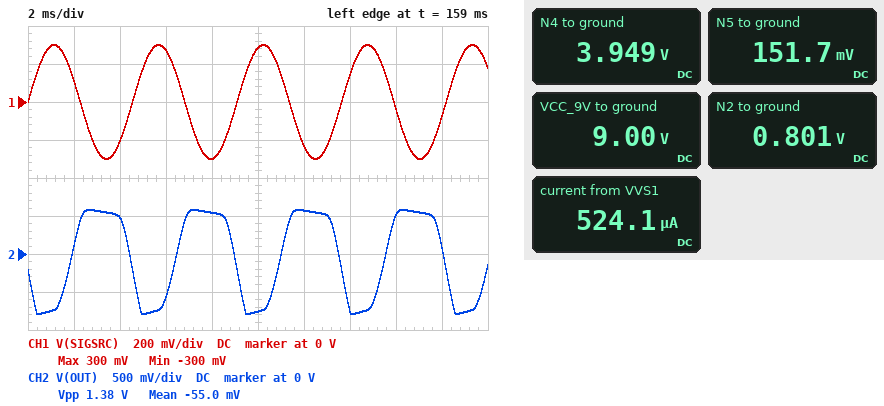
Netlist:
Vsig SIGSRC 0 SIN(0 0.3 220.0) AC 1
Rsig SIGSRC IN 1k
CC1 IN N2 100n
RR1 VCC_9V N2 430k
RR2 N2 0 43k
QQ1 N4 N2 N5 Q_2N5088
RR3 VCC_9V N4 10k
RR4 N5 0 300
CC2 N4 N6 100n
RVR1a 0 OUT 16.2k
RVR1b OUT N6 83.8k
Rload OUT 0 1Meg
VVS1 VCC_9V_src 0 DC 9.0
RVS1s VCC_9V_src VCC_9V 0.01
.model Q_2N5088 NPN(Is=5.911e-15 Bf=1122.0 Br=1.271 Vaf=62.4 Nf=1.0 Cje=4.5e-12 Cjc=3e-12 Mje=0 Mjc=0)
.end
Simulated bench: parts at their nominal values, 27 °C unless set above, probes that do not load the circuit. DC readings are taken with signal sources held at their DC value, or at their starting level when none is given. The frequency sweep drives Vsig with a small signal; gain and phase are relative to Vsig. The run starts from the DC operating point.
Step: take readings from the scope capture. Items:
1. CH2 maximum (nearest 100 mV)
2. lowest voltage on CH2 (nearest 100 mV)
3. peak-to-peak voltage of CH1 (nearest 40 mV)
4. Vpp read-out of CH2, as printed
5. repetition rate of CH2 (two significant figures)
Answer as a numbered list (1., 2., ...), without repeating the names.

1. 600 mV
2. -800 mV
3. 600 mV
4. 1.38 V
5. 220 Hz
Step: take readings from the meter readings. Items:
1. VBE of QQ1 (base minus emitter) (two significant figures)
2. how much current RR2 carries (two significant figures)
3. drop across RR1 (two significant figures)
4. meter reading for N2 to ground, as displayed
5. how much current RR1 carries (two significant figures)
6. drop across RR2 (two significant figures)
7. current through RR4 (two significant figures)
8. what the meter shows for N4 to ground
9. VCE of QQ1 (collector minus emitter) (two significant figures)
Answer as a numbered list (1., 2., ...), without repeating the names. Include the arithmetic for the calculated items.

1. 801 mV - 151.7 mV = 650 mV
2. (801 mV) / 43 kΩ = 19 µA
3. 9 V - 801 mV = 8.2 V
4. 0.801 V
5. (9 V - 801 mV) / 430 kΩ = 19 µA
6. 801 mV = 800 mV
7. (151.7 mV) / 300 Ω = 510 µA
8. 3.949 V
9. 3.949 V - 151.7 mV = 3.8 V
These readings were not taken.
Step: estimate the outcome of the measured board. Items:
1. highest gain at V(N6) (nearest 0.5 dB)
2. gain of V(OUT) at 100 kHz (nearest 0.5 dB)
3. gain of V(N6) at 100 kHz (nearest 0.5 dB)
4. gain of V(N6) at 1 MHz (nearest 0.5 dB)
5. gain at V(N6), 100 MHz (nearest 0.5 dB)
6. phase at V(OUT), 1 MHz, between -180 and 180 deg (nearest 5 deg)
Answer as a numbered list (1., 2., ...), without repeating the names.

1. 28.0 dB
2. 12.0 dB
3. 28.0 dB
4. 26.5 dB
5. -6.5 dB
6. 145 deg
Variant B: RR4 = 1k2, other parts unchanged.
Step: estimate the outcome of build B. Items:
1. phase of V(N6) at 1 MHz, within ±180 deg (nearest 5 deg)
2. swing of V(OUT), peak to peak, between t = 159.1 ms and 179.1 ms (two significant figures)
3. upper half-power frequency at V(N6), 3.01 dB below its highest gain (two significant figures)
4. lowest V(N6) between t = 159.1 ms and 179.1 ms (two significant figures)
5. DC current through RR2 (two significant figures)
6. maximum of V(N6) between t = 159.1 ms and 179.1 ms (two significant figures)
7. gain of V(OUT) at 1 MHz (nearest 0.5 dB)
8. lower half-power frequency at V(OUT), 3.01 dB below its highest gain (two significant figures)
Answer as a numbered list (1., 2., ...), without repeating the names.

1. 160 deg
2. 550 mV
3. 3.2 MHz
4. -1.9 V
5. 19 µA
6. 1.6 V
7. 0 dB
8. 45 Hz
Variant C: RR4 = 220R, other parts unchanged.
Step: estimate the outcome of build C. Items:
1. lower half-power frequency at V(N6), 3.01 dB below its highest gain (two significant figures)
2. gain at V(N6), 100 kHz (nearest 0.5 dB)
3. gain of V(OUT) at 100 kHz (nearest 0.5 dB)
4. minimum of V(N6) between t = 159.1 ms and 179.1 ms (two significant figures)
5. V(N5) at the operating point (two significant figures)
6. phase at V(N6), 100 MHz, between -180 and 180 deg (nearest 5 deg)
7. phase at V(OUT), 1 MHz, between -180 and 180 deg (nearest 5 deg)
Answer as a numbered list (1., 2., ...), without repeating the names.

1. 49 Hz
2. 30.5 dB
3. 14.5 dB
4. -5.2 V
5. 140 mV
6. 60 deg
7. 140 deg
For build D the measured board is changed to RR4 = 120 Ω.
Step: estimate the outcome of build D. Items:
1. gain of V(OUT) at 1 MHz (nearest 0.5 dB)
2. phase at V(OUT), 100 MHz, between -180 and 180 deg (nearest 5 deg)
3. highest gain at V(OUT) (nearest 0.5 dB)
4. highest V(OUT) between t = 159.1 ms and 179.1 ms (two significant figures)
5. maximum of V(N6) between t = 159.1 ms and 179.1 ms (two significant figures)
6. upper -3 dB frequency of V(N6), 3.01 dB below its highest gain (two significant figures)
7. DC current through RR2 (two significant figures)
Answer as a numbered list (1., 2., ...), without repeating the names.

1. 11.0 dB
2. 70 deg
3. 12.5 dB
4. 560 mV
5. 3.5 V
6. 1.7 MHz
7. 18 µA
